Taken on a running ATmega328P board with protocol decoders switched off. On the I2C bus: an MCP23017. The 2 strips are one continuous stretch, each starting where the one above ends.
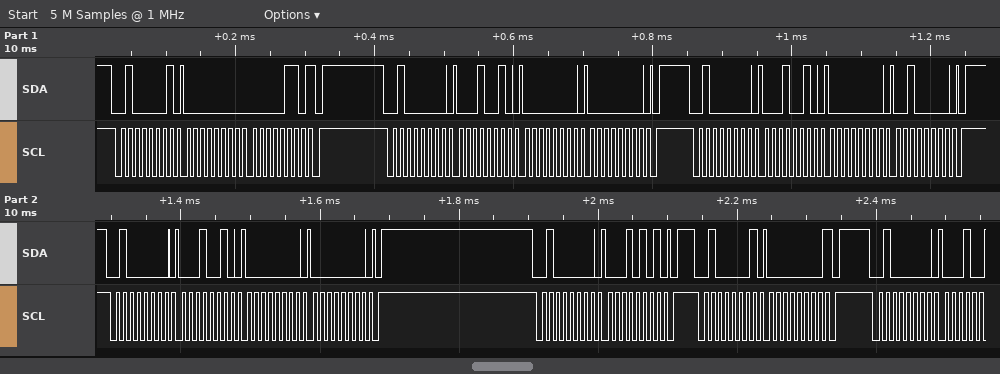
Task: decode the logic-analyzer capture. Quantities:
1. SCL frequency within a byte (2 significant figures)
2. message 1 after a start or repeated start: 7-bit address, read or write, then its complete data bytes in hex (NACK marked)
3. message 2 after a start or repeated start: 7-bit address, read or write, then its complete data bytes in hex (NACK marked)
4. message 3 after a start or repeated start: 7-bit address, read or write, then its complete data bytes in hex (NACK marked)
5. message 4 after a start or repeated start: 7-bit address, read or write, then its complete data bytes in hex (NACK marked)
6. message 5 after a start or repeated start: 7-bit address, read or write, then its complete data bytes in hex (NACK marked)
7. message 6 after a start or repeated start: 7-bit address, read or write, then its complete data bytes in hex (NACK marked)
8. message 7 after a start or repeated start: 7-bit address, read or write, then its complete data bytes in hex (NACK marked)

100 kHz
0x20 read: 00 06 NACK
0x20 write: 12 00 00
0x20 write: 12 00 20
0x20 write: 12 00 00
0x20 write: 15
0x20 read: 00 NACK
0x20 write
